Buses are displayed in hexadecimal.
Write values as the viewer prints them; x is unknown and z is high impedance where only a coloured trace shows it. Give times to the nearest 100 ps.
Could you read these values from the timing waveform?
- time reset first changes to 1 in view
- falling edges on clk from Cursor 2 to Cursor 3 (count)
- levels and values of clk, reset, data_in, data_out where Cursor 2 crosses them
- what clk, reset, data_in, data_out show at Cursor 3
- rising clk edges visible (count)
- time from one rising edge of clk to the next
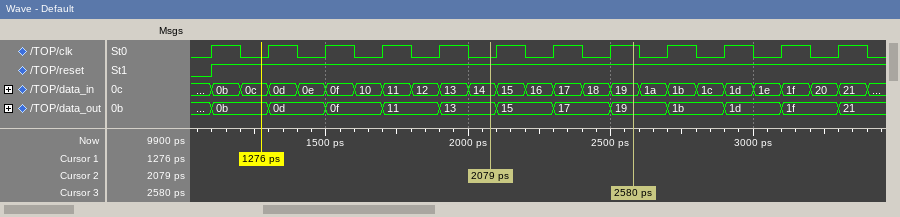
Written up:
1100 ps
2
clk=0, reset=1, data_in=14, data_out=13
clk=1, reset=1, data_in=19, data_out=19
12
200 ps
